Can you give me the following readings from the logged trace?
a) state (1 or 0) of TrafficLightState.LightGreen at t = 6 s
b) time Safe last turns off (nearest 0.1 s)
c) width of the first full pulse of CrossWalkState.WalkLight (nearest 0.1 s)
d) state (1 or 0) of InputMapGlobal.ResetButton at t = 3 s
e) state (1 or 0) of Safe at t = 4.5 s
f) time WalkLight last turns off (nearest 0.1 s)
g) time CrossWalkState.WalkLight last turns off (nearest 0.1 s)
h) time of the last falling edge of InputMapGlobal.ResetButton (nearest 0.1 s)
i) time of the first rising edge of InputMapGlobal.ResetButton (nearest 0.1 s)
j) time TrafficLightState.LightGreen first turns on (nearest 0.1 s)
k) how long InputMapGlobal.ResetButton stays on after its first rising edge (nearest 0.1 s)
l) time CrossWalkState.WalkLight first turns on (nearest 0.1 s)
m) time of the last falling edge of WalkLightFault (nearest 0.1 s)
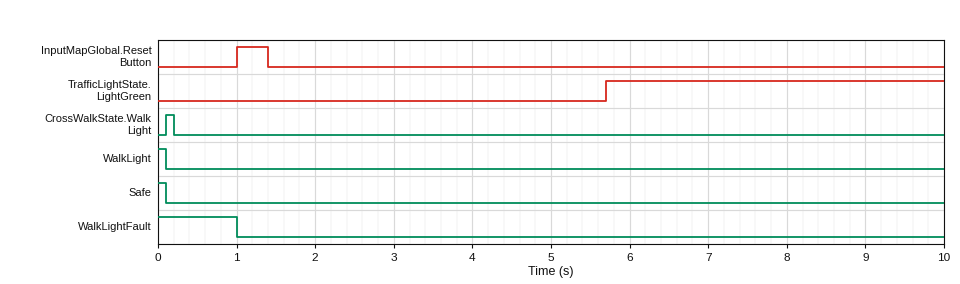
1
0.1 s
0.1 s
0
0
0.1 s
0.2 s
1.4 s
1.0 s
5.7 s
0.4 s
0.1 s
1.0 s
